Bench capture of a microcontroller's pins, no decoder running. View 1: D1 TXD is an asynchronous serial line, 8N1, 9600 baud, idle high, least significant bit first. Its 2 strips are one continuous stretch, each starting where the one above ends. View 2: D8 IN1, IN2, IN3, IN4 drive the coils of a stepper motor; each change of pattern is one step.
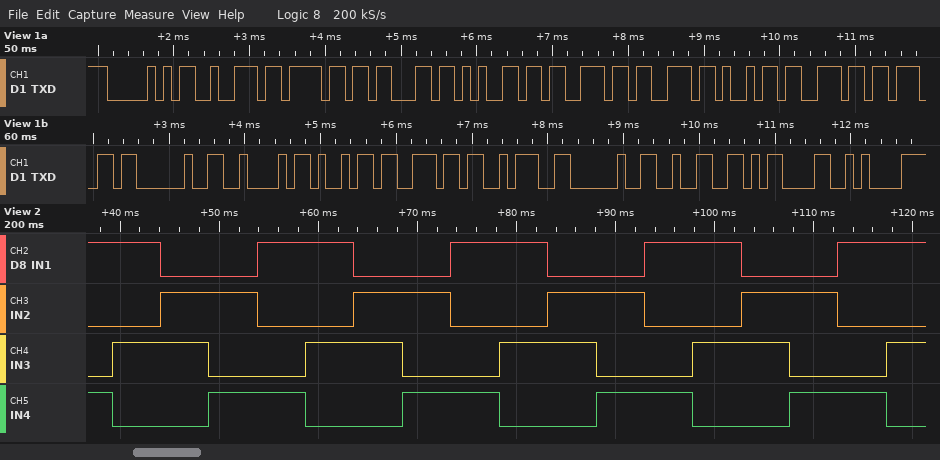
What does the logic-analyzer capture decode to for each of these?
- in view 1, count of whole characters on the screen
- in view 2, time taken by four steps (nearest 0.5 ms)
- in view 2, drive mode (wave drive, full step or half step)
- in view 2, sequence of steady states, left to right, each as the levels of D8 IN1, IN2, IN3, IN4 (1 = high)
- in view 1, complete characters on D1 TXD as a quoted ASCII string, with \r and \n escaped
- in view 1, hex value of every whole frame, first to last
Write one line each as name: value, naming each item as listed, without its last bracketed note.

in view 1, count of whole characters on the screen: 19
in view 2, time taken by four steps: 19.5 ms
in view 2, drive mode: full step
in view 2, sequence of steady states, left to right, each as the levels of D8 IN1, IN2, IN3, IN4: 1001 1010 0110 0101 1001 1010 0110 0101 1001 1010 0110 0101 1001 1010 0110 0101 1001 1010
in view 1, complete characters on D1 TXD as a quoted ASCII string, with \r and \n escaped: "Processing Bin: 2\r\n"
in view 1, hex value of every whole frame, first to last: 0x50 0x72 0x6F 0x63 0x65 0x73 0x73 0x69 0x6E 0x67 0x20 0x42 0x69 0x6E 0x3A 0x20 0x32 0x0D 0x0A
